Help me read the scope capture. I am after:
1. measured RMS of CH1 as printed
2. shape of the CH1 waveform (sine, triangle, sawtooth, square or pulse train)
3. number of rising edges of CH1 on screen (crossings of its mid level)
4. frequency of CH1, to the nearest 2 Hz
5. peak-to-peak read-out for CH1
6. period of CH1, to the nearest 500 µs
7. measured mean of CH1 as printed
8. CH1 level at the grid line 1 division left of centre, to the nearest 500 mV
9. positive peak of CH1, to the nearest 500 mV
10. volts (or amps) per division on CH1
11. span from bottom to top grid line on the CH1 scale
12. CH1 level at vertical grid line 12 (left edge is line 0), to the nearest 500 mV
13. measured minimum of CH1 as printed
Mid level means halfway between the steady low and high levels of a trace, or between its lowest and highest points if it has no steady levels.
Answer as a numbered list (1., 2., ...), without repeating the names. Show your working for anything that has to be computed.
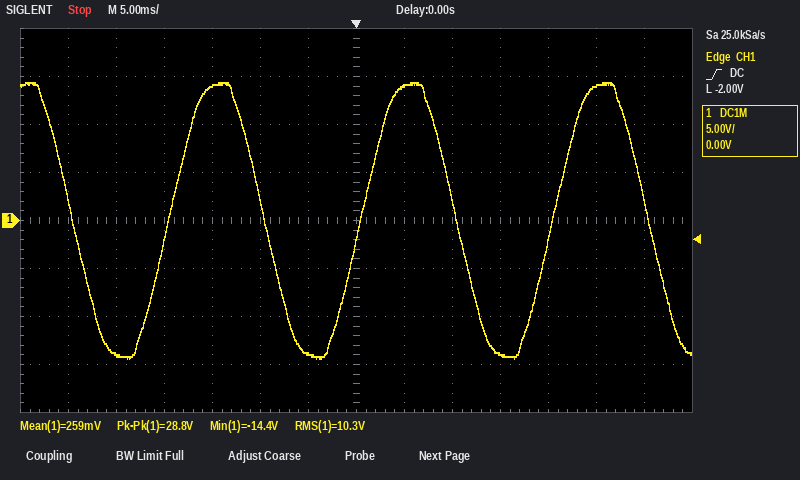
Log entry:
1. 10.3 V
2. sine
3. 3
4. 1 / 20.0 ms ≈ 50 Hz
5. 28.8 V
6. 20.0 ms
7. 259 mV
8. -14.0 V
9. 14.5 V
10. 5 V
11. 40 V
12. 14.0 V
13. -14.4 V
